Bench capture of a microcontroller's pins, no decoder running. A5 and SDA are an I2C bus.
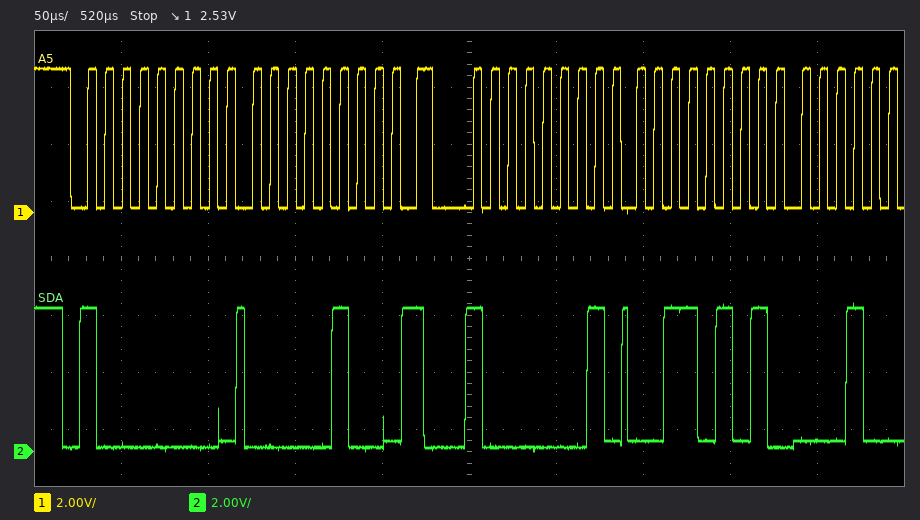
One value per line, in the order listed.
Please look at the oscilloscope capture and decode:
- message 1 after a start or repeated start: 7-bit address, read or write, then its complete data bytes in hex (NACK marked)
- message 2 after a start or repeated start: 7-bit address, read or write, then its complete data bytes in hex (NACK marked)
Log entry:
0x40 write: 04
0x40 read: 35
